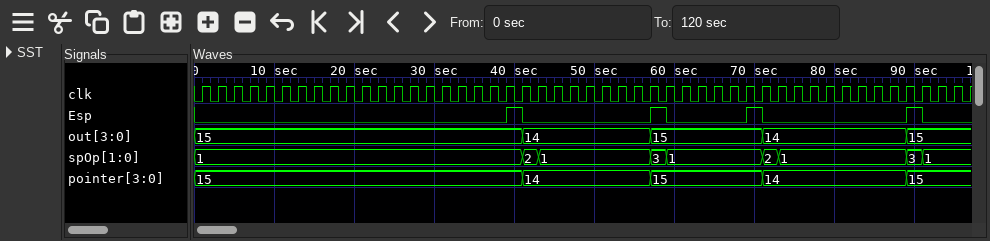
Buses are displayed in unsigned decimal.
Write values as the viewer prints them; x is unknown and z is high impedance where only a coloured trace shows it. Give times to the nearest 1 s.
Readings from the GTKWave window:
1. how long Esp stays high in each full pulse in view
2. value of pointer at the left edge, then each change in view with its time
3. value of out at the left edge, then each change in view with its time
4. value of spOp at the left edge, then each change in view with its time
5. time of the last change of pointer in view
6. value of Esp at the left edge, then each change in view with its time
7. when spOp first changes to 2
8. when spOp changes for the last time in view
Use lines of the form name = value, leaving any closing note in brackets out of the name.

how long Esp stays high in each full pulse in view = 2 s, 2 s, 2 s, 2 s
value of pointer at the left edge, then each change in view with its time = 15, 14 at 41 s, 15 at 57 s, 14 at 71 s, 15 at 89 s
value of out at the left edge, then each change in view with its time = 15, 14 at 41 s, 15 at 57 s, 14 at 71 s, 15 at 89 s
value of spOp at the left edge, then each change in view with its time = 1, 2 at 41 s, 1 at 43 s, 3 at 57 s, 1 at 59 s, 2 at 71 s, 1 at 73 s, 3 at 89 s, 1 at 91 s
time of the last change of pointer in view = 89 s
value of Esp at the left edge, then each change in view with its time = 0, 1 at 39 s, 0 at 41 s, 1 at 57 s, 0 at 59 s, 1 at 69 s, 0 at 71 s, 1 at 89 s, 0 at 91 s
when spOp first changes to 2 = 41 s
when spOp changes for the last time in view = 91 s
